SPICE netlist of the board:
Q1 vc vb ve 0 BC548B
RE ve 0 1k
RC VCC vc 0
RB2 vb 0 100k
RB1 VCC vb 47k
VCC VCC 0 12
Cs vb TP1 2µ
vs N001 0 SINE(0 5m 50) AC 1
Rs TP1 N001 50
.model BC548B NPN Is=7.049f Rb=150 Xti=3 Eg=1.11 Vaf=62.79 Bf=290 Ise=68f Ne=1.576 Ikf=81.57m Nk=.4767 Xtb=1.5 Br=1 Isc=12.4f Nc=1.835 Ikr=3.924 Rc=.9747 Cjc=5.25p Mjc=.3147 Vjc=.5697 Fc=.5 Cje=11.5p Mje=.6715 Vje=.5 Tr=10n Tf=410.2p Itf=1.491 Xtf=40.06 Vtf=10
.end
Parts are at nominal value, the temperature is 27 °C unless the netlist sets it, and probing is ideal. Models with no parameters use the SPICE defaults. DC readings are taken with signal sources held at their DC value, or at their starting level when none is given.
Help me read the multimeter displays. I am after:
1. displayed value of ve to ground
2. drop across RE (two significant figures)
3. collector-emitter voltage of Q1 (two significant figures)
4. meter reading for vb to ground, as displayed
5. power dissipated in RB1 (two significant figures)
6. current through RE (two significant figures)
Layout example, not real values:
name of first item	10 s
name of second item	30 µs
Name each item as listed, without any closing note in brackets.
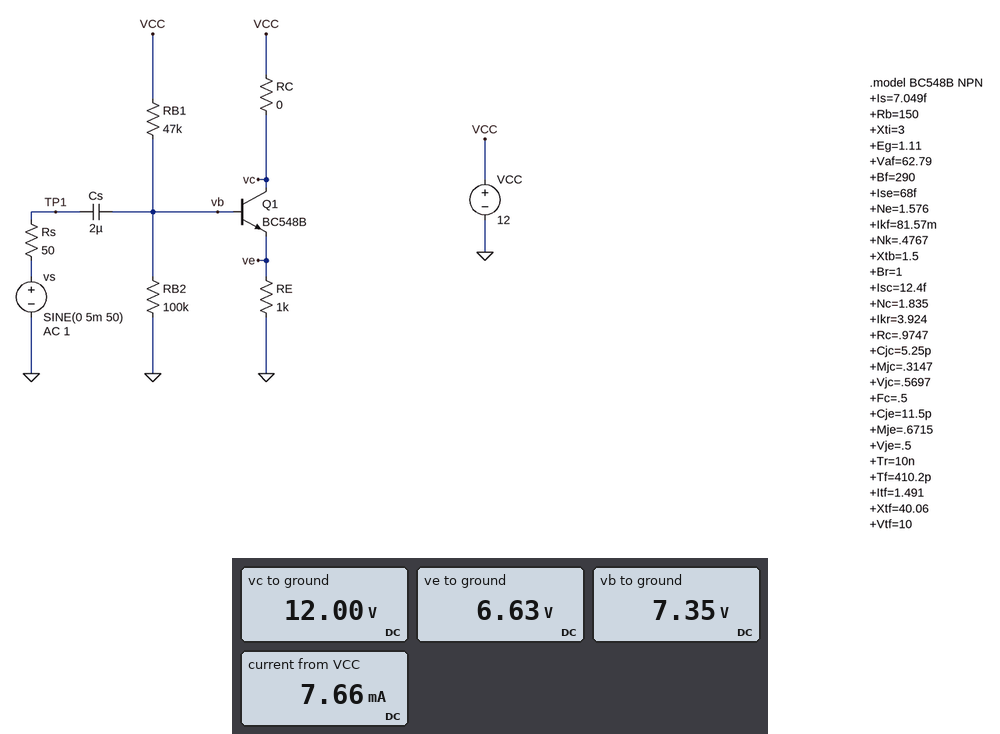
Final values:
displayed value of ve to ground	6.63 V
drop across RE	6.6 V
collector-emitter voltage of Q1	5.4 V
meter reading for vb to ground, as displayed	7.35 V
power dissipated in RB1	460 µW
current through RE	6.6 mA
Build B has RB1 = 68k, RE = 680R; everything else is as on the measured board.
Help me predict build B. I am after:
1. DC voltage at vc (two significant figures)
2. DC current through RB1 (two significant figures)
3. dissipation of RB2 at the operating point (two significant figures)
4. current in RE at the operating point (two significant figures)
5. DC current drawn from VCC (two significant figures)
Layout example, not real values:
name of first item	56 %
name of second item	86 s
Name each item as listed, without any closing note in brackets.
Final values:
DC voltage at vc	12 V
DC current through RB1	89 µA
dissipation of RB2 at the operating point	360 µW
current in RE at the operating point	7.7 mA
DC current drawn from VCC	9.7 mA
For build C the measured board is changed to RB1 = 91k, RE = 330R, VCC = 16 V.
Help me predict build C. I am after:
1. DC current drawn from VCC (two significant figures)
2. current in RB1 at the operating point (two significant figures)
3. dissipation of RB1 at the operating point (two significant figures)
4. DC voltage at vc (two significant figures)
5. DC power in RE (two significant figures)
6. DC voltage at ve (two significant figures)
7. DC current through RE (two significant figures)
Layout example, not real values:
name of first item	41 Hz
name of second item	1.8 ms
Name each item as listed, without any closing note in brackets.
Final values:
DC current drawn from VCC	14 mA
current in RB1 at the operating point	110 µA
dissipation of RB1 at the operating point	1.2 mW
DC voltage at vc	16 V
DC power in RE	75 mW
DC voltage at ve	5.0 V
DC current through RE	15 mA
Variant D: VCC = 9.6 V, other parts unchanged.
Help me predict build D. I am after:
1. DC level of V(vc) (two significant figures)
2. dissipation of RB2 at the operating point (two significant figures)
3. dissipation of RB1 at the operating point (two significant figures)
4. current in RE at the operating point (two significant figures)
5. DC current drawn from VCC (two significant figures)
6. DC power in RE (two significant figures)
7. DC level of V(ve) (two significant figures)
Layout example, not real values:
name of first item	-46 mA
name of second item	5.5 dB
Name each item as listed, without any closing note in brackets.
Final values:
DC level of V(vc)	9.6 V
dissipation of RB2 at the operating point	350 µW
dissipation of RB1 at the operating point	290 µW
current in RE at the operating point	5.2 mA
DC current drawn from VCC	5.7 mA
DC power in RE	27 mW
DC level of V(ve)	5.2 V
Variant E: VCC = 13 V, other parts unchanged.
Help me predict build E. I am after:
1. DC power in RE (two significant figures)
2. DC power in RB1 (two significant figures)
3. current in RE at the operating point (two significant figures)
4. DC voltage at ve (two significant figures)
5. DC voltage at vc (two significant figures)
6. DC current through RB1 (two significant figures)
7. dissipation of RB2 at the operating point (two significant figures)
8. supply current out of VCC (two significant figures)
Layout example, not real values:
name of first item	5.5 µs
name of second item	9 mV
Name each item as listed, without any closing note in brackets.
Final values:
DC power in RE	52 mW
DC power in RB1	540 µW
current in RE at the operating point	7.2 mA
DC voltage at ve	7.2 V
DC voltage at vc	13 V
DC current through RB1	110 µA
dissipation of RB2 at the operating point	630 µW
supply current out of VCC	7.6 mA
